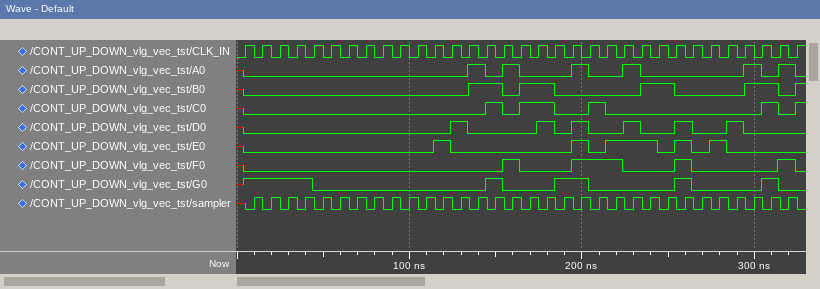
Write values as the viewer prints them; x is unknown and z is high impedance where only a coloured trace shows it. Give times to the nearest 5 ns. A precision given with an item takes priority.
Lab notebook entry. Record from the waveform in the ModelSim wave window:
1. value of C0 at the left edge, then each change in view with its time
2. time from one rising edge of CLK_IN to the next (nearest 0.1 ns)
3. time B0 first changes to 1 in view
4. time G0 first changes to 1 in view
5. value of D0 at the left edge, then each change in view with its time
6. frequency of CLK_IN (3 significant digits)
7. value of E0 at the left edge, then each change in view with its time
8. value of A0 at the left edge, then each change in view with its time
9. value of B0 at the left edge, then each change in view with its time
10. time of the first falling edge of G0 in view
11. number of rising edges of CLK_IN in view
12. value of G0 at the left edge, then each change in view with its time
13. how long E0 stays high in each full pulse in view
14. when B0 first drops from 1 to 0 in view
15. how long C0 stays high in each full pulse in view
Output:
x, 0 at 5 ns, 1 at 145 ns, 0 at 155 ns, 1 at 165 ns, 0 at 185 ns, 1 at 205 ns, 0 at 215 ns, 1 at 305 ns, 0 at 315 ns, 1 at 325 ns
10 ns
135 ns
5 ns
x, 0 at 5 ns, 1 at 125 ns, 0 at 135 ns, 1 at 175 ns, 0 at 185 ns, 1 at 195 ns, 0 at 205 ns, 1 at 225 ns, 0 at 235 ns, 1 at 255 ns, 0 at 265 ns, 1 at 285 ns, 0 at 295 ns
100 MHz
x, 0 at 5 ns, 1 at 115 ns, 0 at 125 ns, 1 at 195 ns, 0 at 205 ns, 1 at 215 ns, 0 at 245 ns, 1 at 255 ns, 0 at 265 ns, 1 at 275 ns, 0 at 285 ns
x, 0 at 5 ns, 1 at 135 ns, 0 at 145 ns, 1 at 155 ns, 0 at 165 ns, 1 at 195 ns, 0 at 205 ns, 1 at 225 ns, 0 at 235 ns, 1 at 295 ns, 0 at 305 ns, 1 at 315 ns, 0 at 325 ns
x, 0 at 5 ns, 1 at 135 ns, 0 at 155 ns, 1 at 165 ns, 0 at 185 ns, 1 at 235 ns, 0 at 255 ns, 1 at 295 ns, 0 at 315 ns, 1 at 325 ns
45 ns
33
x, 1 at 5 ns, 0 at 45 ns, 1 at 145 ns, 0 at 155 ns, 1 at 185 ns, 0 at 205 ns, 1 at 255 ns, 0 at 265 ns, 1 at 305 ns, 0 at 315 ns
10 ns, 10 ns, 30 ns, 10 ns, 10 ns
155 ns
10 ns, 20 ns, 10 ns, 10 ns
